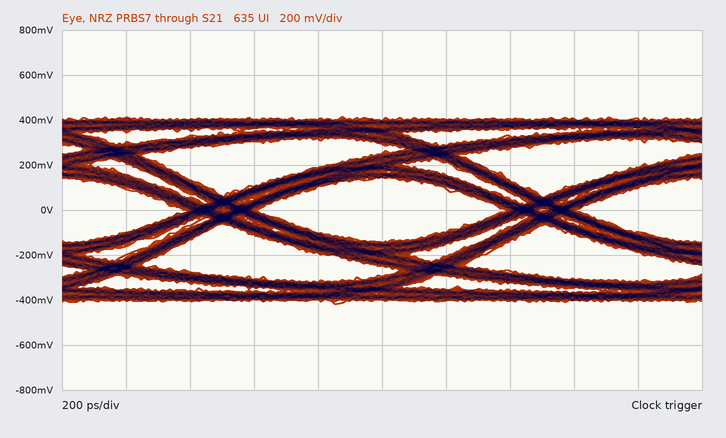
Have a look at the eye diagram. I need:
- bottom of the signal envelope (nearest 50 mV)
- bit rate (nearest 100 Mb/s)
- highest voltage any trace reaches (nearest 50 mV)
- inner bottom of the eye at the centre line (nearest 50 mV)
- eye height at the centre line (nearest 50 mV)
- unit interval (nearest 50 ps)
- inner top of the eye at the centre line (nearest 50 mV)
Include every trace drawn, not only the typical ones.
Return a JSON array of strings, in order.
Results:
["-400 mV", "1.0 Gb/s", "400 mV", "-150 mV", "300 mV", "1.00 ns", "150 mV"]
